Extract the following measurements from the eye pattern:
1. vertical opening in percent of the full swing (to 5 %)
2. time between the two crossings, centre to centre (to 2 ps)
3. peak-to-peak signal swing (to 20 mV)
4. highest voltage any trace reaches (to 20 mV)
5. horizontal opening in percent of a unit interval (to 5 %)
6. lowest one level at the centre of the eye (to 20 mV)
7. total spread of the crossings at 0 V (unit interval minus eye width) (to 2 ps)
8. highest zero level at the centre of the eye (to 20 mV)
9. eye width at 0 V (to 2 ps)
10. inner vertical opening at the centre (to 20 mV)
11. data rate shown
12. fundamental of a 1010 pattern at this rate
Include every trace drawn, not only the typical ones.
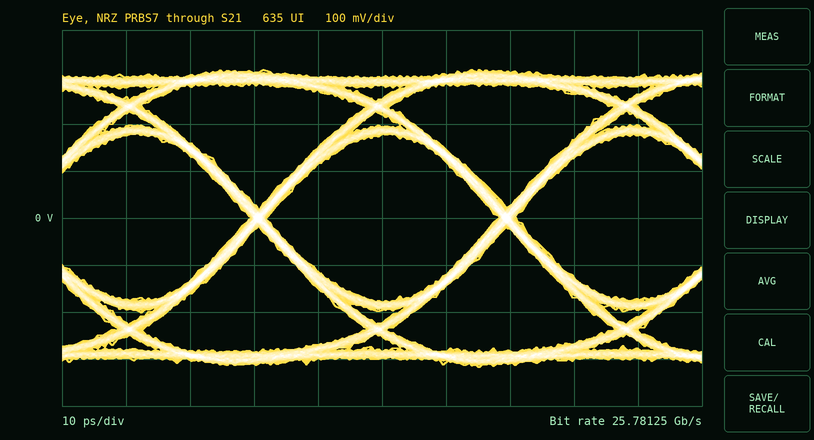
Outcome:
55 %
38 ps
640 mV
320 mV
95 %
180 mV
2 ps
-180 mV
36 ps
360 mV
25.78125 Gb/s
12.89062 GHz
